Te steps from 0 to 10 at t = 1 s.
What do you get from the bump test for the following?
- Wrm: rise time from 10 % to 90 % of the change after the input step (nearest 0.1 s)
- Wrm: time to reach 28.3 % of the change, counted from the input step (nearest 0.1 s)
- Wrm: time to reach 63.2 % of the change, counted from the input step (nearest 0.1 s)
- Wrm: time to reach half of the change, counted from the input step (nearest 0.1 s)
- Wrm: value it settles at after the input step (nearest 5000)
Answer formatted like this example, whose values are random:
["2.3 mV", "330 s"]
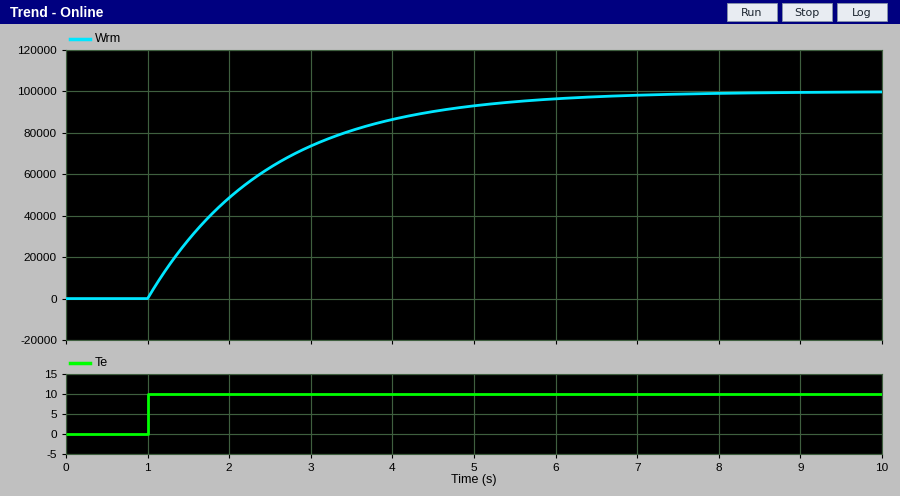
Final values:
["3.3 s", "0.5 s", "1.5 s", "1.0 s", "100000"]
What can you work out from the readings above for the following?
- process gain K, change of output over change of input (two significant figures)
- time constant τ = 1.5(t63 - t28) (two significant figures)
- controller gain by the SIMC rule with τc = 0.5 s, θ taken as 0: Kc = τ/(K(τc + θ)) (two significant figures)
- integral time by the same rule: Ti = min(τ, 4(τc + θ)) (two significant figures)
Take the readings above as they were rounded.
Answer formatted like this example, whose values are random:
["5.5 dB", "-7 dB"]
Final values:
["10000", "1.5 s", "0.00030", "1.5 s"]
